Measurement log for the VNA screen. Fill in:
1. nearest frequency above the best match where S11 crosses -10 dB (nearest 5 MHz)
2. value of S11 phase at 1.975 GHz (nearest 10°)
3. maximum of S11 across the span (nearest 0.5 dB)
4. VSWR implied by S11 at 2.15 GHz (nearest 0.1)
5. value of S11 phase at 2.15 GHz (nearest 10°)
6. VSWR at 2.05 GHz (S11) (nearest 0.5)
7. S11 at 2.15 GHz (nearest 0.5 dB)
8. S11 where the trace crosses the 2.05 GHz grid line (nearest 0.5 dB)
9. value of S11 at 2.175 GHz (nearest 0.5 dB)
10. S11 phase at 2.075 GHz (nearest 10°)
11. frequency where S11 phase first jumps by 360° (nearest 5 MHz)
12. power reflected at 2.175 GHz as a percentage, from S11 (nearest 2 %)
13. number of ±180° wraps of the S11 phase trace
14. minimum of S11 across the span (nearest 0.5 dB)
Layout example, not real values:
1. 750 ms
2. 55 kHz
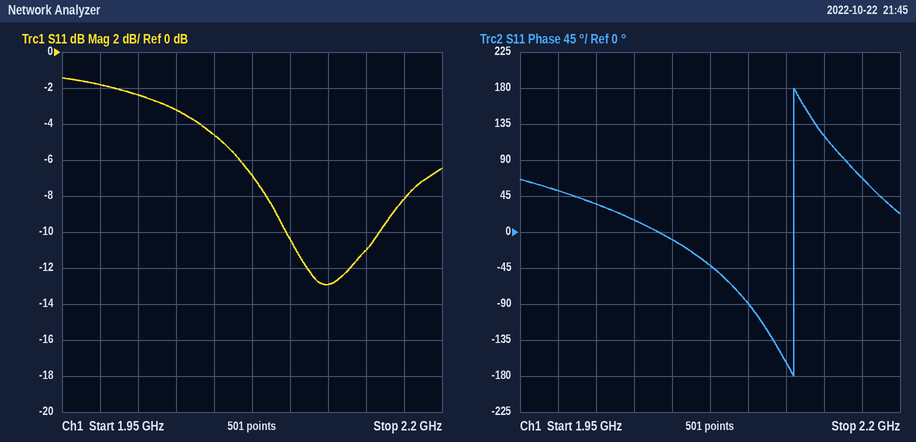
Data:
1. 2.160 GHz
2. 50°
3. -1.5 dB
4. 1.8
5. 120°
6. 4.0
7. -11.0 dB
8. -4.5 dB
9. -8.0 dB
10. -40°
11. 2.130 GHz
12. 16 %
13. 1
14. -13.0 dB
